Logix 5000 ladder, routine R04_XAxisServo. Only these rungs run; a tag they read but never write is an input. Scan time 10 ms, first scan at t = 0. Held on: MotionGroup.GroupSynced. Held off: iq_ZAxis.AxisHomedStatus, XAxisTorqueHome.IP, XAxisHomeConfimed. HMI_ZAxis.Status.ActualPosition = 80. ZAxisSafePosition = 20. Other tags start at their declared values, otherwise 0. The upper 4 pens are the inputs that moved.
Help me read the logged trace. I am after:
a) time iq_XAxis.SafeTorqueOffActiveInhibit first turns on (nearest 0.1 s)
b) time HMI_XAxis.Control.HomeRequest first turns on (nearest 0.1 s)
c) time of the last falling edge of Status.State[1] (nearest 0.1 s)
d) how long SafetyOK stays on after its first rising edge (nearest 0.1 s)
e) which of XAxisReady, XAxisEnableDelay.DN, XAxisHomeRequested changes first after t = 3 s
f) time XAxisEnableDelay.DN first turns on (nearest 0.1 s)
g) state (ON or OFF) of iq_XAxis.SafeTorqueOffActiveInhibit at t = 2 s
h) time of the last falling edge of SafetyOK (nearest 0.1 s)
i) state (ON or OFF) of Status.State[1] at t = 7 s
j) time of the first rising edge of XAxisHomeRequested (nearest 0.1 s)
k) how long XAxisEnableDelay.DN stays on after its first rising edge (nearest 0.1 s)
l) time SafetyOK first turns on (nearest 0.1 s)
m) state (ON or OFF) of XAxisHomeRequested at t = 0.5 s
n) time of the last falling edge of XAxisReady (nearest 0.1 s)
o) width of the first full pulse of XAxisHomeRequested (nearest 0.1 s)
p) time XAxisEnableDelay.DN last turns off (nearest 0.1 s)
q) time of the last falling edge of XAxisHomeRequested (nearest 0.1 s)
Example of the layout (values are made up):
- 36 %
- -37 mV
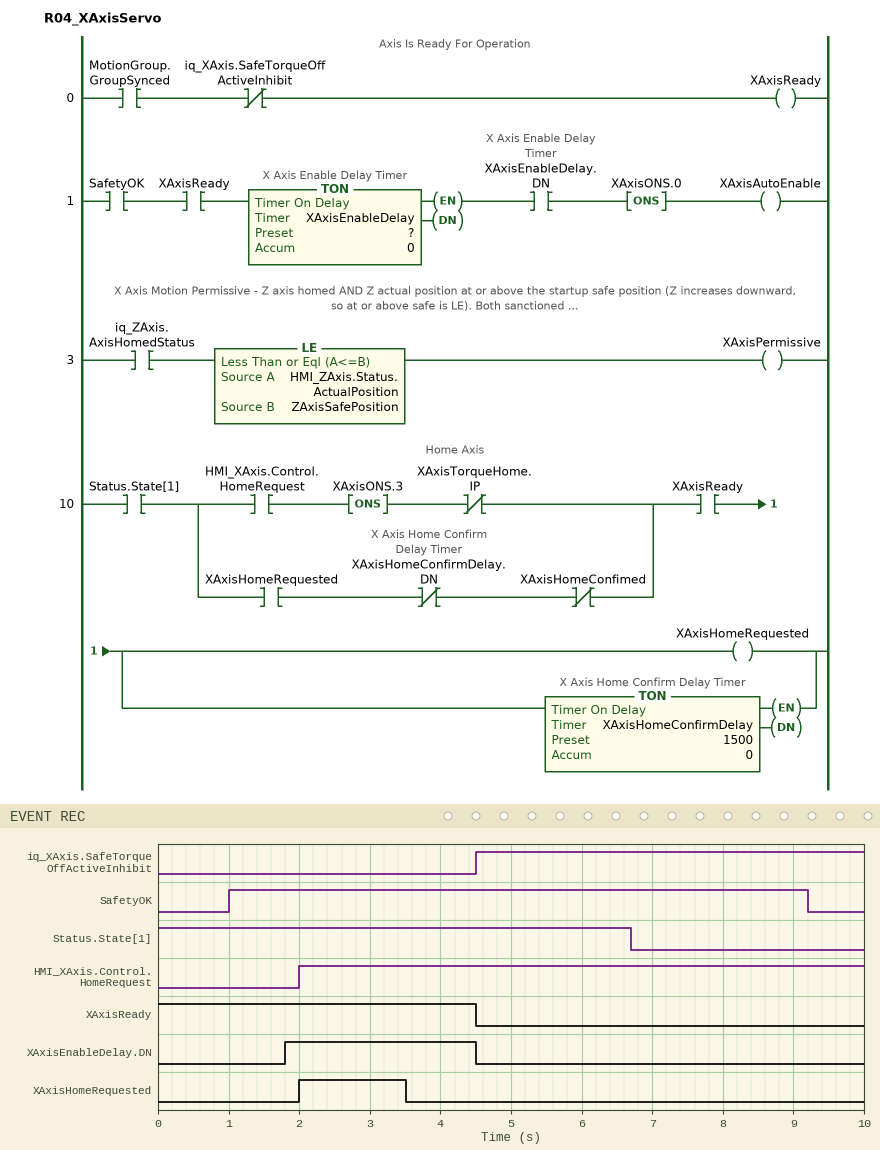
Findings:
- 4.5 s
- 2.0 s
- 6.7 s
- 8.2 s
- XAxisHomeRequested
- 1.8 s
- OFF
- 9.2 s
- OFF
- 2.0 s
- 2.7 s
- 1.0 s
- OFF
- 4.5 s
- 1.5 s
- 4.5 s
- 3.5 s
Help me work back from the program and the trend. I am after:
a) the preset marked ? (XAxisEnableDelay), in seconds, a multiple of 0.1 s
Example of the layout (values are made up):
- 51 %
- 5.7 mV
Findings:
- 0.8 s
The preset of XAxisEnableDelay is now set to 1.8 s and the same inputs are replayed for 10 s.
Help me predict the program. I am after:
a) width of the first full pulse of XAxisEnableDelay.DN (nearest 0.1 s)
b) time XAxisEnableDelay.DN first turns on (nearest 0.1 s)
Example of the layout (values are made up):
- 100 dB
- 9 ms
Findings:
- 1.7 s
- 2.8 s
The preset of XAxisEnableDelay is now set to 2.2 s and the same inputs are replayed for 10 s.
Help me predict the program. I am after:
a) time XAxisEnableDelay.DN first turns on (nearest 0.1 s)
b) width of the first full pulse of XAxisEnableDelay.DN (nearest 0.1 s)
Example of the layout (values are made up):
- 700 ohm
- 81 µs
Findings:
- 3.2 s
- 1.3 s
